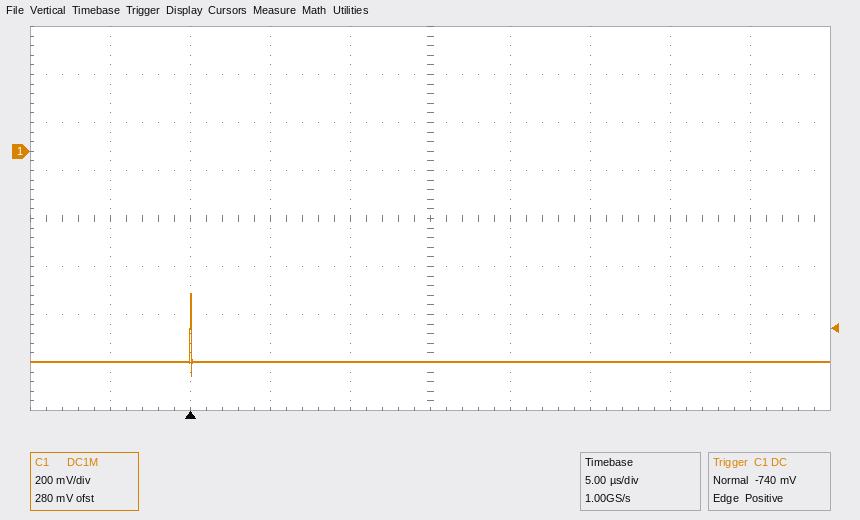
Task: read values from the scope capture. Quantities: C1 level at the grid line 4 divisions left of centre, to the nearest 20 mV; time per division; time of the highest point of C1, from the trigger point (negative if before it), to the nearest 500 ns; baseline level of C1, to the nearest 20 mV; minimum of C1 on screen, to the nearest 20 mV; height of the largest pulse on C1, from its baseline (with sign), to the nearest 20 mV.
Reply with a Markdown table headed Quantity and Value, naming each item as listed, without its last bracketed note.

| Quantity | Value |
|---|---|
| C1 level at the grid line 4 divisions left of centre, to the nearest 20 mV | -880 mV |
| time per division | 5 µs |
| time of the highest point of C1, from the trigger point (negative if before it), to the nearest 500 ns | 0.0 µs |
| baseline level of C1, to the nearest 20 mV | -880 mV |
| minimum of C1 on screen, to the nearest 20 mV | -940 mV |
| height of the largest pulse on C1, from its baseline (with sign), to the nearest 20 mV | +280 mV |
